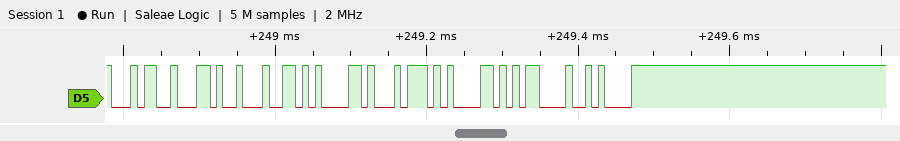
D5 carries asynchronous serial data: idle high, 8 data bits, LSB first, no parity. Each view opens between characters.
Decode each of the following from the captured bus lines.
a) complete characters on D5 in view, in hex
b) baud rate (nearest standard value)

34, 2C, 64, 61, 74, 61, 0D, 0A
115200 baud
